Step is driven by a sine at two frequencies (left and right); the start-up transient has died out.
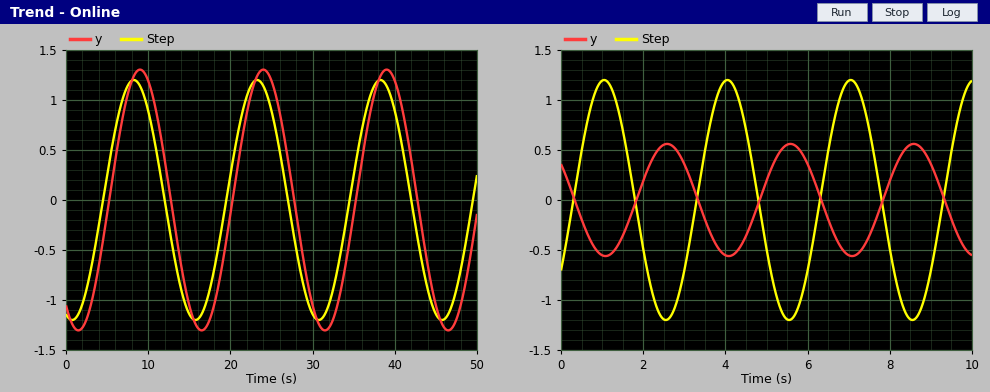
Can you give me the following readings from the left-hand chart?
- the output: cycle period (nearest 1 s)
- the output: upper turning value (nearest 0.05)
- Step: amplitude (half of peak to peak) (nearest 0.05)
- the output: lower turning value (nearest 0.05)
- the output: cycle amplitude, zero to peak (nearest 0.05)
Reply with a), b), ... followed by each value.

a) 15 s
b) 1.30
c) 1.20
d) -1.30
e) 1.30
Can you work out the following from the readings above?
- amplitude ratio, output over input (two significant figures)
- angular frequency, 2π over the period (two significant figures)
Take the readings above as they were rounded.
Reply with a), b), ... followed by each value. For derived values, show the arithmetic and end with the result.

a) 1.3 / 1.2 = 1.1
b) 2π / 15 = 0.42 rad/s
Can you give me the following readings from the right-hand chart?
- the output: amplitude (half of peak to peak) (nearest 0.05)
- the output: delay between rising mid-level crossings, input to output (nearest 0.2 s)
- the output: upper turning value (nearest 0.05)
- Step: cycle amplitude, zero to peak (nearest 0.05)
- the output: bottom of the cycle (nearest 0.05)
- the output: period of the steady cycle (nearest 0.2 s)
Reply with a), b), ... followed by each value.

a) 0.55
b) 1.6 s
c) 0.55
d) 1.20
e) -0.55
f) 3.0 s
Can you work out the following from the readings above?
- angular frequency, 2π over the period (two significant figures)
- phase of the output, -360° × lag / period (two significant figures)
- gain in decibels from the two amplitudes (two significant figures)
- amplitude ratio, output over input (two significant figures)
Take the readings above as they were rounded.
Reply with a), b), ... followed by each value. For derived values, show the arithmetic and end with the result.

a) 2π / 3 = 2.1 rad/s
b) -360 × 1.6 / 3 = -190°
c) 20 log10(0.55 / 1.2) = -6.8 dB
d) 0.55 / 1.2 = 0.46
